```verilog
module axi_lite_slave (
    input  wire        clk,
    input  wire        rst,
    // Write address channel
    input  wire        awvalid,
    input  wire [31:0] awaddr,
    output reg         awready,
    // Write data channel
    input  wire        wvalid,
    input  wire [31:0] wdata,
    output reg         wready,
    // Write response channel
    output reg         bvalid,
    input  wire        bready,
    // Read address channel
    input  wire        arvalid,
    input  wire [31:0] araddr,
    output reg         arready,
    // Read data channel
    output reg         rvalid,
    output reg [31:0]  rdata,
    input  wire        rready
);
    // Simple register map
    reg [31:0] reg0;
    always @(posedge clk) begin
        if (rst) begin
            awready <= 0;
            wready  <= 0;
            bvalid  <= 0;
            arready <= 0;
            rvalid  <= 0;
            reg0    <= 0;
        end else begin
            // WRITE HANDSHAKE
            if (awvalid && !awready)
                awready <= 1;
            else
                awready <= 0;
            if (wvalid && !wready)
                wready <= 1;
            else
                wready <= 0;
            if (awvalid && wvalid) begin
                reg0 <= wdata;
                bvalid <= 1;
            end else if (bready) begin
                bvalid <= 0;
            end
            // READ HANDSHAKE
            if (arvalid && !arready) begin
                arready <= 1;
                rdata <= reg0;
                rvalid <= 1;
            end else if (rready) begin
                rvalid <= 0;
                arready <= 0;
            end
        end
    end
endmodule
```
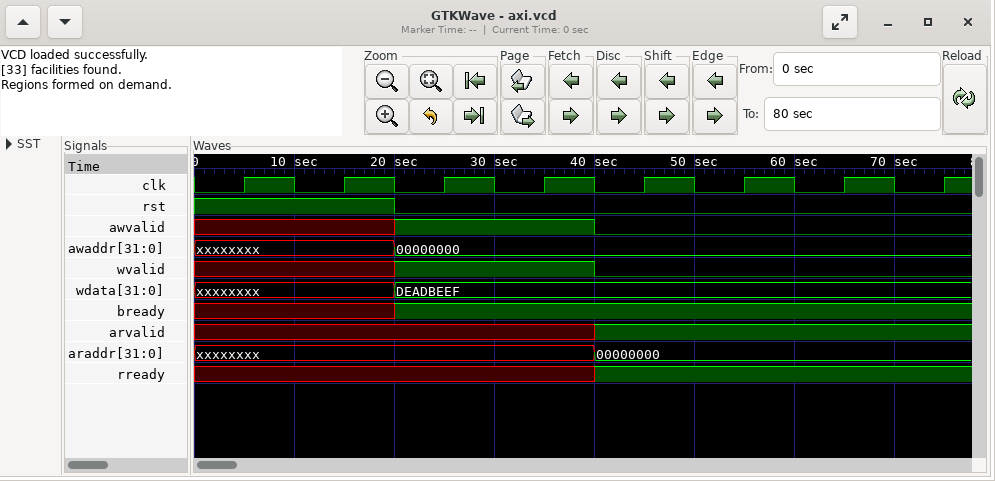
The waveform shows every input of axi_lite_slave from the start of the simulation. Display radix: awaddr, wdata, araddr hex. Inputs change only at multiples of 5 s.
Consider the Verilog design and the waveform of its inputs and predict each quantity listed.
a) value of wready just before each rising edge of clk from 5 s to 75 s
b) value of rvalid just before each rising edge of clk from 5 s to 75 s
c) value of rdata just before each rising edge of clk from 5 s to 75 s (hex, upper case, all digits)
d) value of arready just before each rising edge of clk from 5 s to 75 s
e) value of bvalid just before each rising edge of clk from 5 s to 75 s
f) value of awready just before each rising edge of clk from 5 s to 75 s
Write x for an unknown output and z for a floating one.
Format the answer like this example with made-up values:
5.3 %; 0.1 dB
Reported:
x 0 0 1 0 0 0 0; x 0 0 0 0 1 0 1; x, x, x, x, x, DEADBEEF, DEADBEEF, DEADBEEF; x 0 0 0 0 1 0 1; x 0 0 1 1 0 0 0; x 0 0 1 0 0 0 0
